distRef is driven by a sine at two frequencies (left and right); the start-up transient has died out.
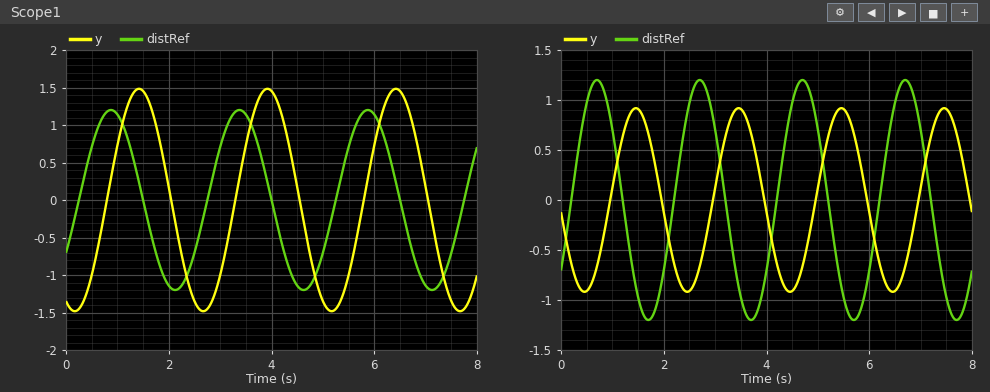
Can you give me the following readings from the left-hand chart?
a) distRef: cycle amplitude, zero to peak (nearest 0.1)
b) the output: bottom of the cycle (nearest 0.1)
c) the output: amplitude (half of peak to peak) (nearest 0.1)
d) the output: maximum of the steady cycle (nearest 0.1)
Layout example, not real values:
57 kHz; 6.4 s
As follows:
1.2; -1.5; 1.5; 1.5
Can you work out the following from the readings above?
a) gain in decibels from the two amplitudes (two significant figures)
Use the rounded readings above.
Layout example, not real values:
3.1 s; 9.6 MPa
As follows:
1.9 dB
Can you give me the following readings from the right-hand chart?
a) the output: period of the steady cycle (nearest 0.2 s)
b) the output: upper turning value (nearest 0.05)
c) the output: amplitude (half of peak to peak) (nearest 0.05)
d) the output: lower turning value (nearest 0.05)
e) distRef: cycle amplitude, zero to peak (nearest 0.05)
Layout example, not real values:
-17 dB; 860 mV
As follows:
2.0 s; 0.90; 0.90; -0.90; 1.20
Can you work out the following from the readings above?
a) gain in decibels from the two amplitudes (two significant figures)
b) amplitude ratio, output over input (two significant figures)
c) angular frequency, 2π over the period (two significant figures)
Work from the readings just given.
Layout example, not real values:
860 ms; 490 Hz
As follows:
-2.5 dB; 0.75; 3.1 rad/s
